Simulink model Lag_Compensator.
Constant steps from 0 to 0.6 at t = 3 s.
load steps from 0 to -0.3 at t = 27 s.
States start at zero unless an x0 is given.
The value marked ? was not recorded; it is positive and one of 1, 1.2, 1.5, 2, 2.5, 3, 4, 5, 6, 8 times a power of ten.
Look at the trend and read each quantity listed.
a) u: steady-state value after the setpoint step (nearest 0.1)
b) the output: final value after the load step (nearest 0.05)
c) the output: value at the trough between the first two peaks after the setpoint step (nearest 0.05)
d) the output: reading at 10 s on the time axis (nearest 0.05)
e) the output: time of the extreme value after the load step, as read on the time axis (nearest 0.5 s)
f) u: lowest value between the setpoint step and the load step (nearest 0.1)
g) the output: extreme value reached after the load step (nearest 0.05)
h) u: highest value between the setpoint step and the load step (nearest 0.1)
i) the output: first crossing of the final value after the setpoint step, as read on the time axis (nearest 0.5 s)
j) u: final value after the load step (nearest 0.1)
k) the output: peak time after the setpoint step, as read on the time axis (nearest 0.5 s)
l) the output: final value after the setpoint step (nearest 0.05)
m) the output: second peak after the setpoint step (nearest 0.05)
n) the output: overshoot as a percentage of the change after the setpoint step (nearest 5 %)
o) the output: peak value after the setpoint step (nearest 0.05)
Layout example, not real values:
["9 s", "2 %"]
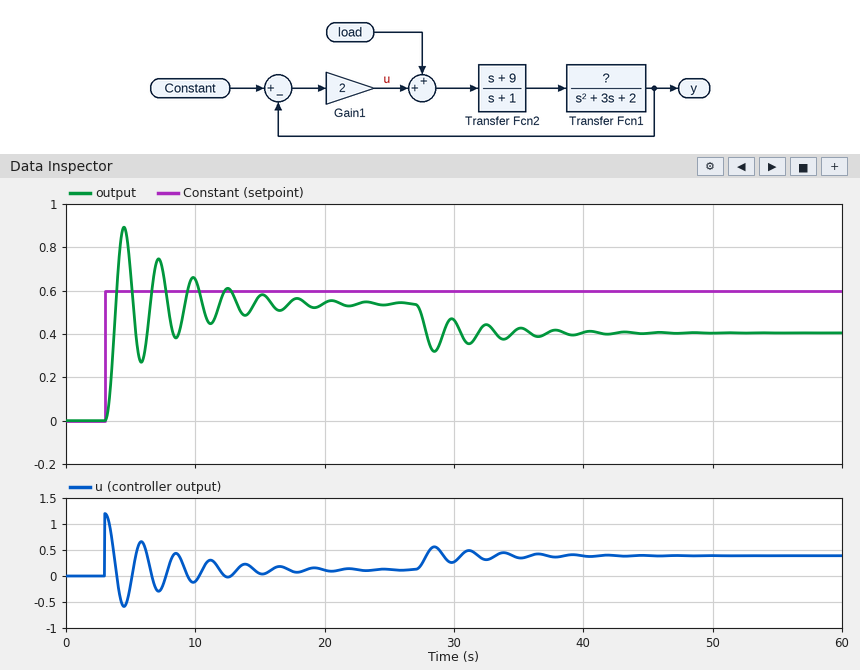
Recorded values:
["0.1", "0.40", "0.25", "0.65", "28.5 s", "-0.6", "0.30", "1.2", "4.0 s", "0.4", "4.5 s", "0.55", "0.75", "65 %", "0.90"]
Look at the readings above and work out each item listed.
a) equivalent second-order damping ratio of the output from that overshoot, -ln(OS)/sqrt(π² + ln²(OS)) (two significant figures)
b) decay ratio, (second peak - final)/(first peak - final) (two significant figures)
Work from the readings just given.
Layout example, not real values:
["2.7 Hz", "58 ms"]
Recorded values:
["0.14", "0.57"]
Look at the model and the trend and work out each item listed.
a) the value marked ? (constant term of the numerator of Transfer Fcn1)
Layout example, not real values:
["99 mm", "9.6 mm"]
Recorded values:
["1"]
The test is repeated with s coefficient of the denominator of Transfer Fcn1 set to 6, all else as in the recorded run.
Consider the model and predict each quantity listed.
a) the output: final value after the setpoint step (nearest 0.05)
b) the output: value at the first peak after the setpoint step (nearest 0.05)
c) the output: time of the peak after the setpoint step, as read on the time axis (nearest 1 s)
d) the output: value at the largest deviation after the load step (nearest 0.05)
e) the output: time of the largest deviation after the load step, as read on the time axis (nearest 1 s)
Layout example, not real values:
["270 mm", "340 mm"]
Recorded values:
["0.55", "0.75", "5 s", "0.35", "29 s"]
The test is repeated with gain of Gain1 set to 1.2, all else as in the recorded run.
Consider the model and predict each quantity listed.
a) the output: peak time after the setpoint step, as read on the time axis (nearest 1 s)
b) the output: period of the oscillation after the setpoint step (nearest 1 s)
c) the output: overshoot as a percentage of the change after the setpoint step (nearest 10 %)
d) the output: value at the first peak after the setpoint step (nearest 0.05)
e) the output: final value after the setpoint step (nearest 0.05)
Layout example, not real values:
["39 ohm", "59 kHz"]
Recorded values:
["5 s", "3 s", "50 %", "0.75", "0.50"]
